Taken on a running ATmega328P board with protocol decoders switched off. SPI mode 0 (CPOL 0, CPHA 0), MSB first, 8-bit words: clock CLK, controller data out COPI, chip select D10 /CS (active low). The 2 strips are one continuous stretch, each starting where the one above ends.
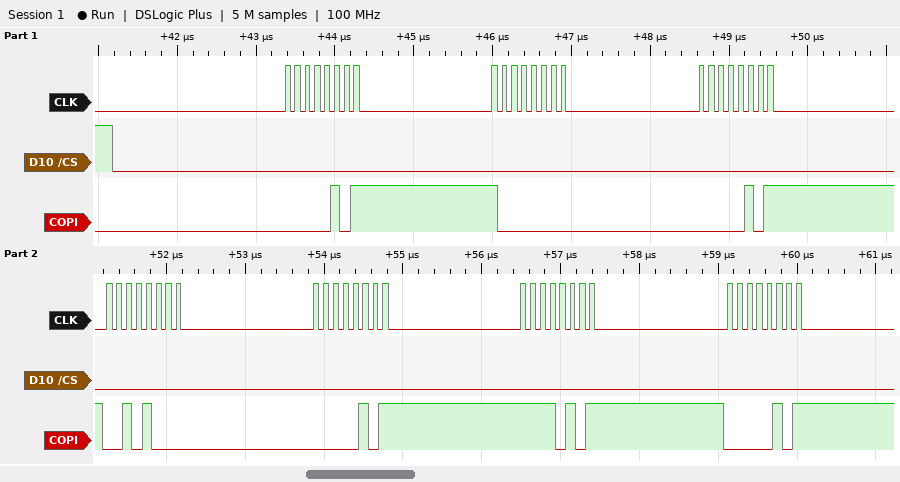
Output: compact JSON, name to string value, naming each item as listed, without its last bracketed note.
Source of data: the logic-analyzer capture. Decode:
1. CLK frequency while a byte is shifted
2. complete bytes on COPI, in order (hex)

{"CLK frequency while a byte is shifted": "8 MHz", "complete bytes on COPI, in order": "0x05 0x80 0x05 0x28 0x05 0xF5 0x05"}
